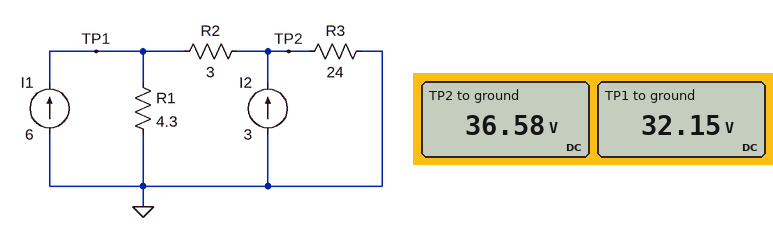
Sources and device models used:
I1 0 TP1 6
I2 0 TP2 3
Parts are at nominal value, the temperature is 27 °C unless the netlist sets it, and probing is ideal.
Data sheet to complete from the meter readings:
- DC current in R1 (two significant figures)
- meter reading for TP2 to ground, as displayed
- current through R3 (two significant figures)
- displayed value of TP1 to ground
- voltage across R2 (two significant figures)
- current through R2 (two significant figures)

7.5 A
36.58 V
1.5 A
32.15 V
4.4 V
1.5 A
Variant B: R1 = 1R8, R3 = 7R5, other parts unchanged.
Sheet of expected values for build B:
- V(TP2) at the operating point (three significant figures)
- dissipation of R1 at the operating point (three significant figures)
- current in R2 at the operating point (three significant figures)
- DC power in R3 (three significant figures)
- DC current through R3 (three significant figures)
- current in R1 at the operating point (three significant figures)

15.4 V
87.0 W
951 mA
31.5 W
2.05 A
6.95 A
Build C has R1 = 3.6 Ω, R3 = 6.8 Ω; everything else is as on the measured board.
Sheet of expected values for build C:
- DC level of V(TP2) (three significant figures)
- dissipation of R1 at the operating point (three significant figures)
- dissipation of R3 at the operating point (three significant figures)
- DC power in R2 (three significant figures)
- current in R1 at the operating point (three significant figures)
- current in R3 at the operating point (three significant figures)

21.0 V
126 W
64.9 W
24.1 mW
5.91 A
3.09 A
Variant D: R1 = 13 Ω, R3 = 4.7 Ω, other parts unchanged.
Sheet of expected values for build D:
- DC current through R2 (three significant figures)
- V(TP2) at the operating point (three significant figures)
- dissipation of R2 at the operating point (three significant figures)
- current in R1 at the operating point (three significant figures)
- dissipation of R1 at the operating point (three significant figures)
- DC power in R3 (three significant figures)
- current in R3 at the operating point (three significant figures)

3.09 A
28.6 V
28.6 W
2.91 A
110 W
174 W
6.09 A
